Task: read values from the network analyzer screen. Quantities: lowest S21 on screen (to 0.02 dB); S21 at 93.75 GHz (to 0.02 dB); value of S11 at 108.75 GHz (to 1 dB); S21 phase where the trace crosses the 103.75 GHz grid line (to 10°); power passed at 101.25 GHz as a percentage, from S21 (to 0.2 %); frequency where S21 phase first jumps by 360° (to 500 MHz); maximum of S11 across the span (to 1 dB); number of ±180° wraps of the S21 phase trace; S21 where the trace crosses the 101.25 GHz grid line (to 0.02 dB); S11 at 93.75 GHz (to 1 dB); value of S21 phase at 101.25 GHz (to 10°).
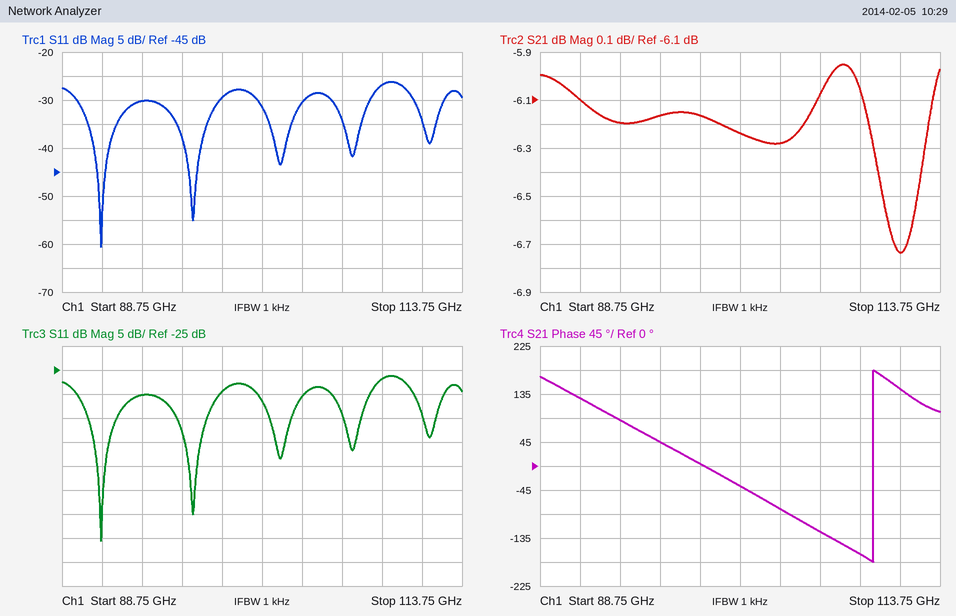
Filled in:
-6.74 dB
-6.20 dB
-27 dB
-80°
23.8 %
109.5 GHz
-26 dB
1
-6.24 dB
-30 dB
-40°
